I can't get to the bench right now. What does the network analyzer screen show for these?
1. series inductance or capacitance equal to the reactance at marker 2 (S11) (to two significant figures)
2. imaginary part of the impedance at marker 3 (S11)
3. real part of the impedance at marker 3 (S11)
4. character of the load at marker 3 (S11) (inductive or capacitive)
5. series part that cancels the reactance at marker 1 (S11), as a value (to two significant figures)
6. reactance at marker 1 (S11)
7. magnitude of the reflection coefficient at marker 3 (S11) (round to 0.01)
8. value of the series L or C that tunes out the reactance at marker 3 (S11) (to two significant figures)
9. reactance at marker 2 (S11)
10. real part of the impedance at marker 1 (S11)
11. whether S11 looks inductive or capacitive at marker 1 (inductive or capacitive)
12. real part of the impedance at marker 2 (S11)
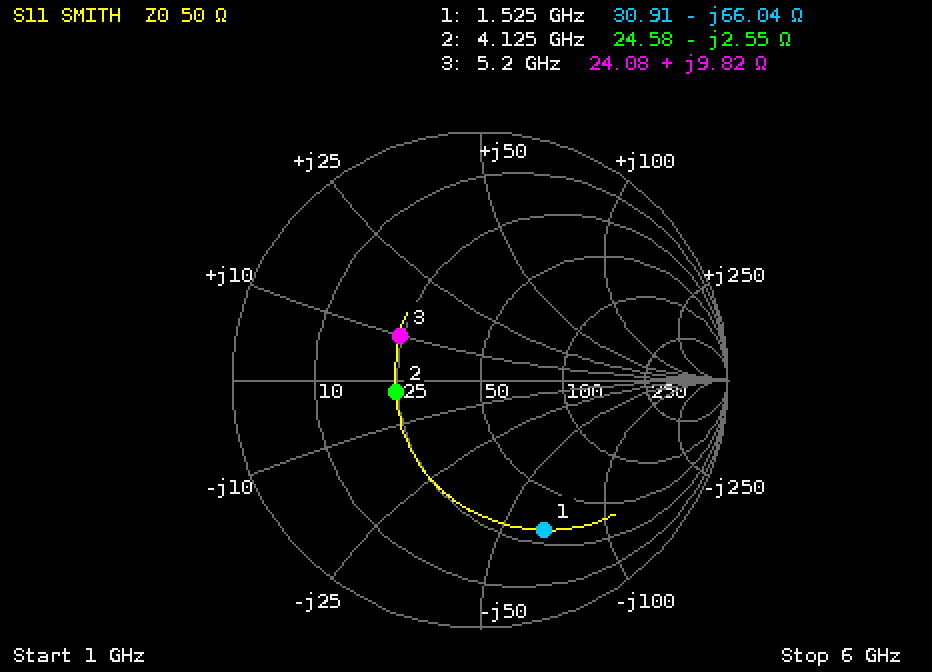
15 pF
+9.82 Ω
24.08 Ω
inductive
6.9 nH
-66.04 Ω
0.37
3.1 pF
-2.55 Ω
30.91 Ω
capacitive
24.58 Ω
